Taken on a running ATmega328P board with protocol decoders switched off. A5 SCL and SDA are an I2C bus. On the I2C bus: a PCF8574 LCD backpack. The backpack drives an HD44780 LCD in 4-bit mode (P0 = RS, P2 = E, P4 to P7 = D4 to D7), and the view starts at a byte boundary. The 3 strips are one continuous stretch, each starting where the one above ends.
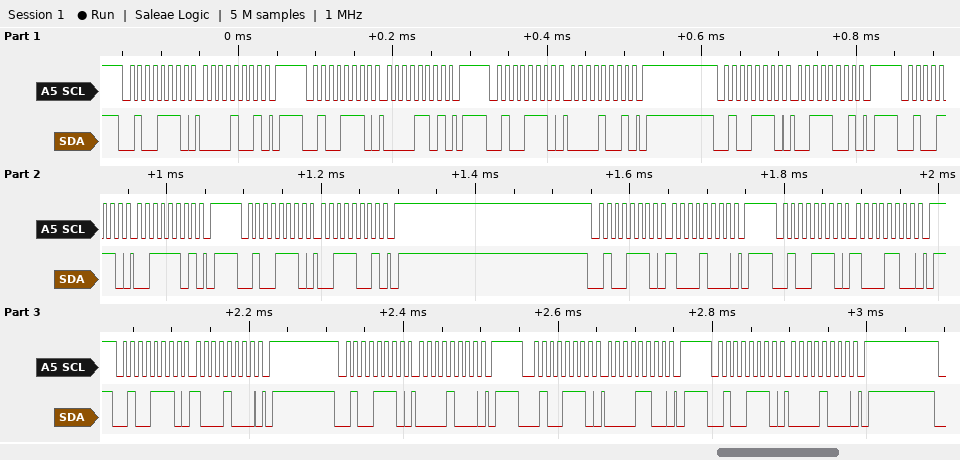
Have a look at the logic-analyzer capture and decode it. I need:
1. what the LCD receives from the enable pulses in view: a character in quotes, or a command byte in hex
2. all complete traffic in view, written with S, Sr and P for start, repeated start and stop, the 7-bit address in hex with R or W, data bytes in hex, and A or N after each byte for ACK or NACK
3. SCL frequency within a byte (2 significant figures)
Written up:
data 0x03 0x80
S 27W A 09 A P S 27W A 0D A P S 27W A 09 A P S 27W A 39 A P S 27W A 3D A P S 27W A 39 A P S 27W A 88 A P S 27W A 8C A P S 27W A 88 A P S 27W A 08 A P S 27W A 0C A P S 27W A 08 A P
100 kHz
